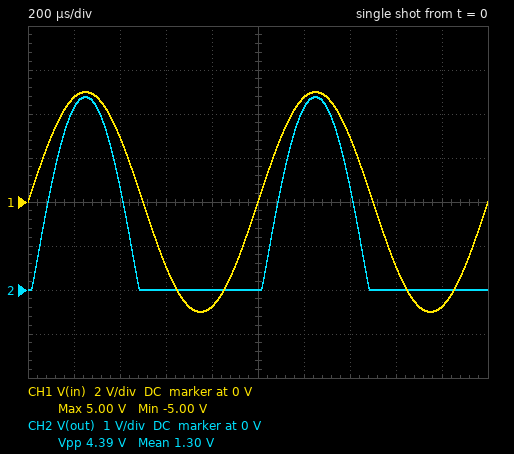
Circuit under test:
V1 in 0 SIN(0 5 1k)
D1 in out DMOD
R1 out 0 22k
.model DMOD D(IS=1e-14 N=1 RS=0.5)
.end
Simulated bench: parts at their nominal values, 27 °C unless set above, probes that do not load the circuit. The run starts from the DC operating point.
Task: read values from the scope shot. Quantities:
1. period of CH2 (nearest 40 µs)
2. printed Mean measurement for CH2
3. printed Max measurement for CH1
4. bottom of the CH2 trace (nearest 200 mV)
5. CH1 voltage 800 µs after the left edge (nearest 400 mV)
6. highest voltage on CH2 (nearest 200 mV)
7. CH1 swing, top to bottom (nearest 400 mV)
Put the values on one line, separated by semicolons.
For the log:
1.00 ms; 1.30 V; 5.00 V; 0 V; -4.8 V; 4.4 V; 10.0 V
